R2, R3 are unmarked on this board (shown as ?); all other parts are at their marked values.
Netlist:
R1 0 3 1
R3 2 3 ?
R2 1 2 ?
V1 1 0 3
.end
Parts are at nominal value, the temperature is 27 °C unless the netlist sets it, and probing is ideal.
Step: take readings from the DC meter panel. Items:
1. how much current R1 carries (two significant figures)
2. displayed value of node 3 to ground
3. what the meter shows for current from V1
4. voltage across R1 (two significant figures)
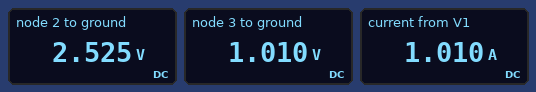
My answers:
1.0 A
1.010 V
1.010 A
1.0 V
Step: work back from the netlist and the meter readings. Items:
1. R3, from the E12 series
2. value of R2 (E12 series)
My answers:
1.5 Ω
0.47 Ω
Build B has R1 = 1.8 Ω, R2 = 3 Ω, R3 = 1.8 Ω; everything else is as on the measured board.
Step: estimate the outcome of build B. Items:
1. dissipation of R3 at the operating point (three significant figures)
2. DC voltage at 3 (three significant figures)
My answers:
372 mW
818 mV
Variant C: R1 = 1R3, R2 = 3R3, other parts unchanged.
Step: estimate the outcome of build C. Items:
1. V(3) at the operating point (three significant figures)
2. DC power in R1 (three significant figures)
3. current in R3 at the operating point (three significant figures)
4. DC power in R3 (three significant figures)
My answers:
639 mV
314 mW
492 mA
363 mW
